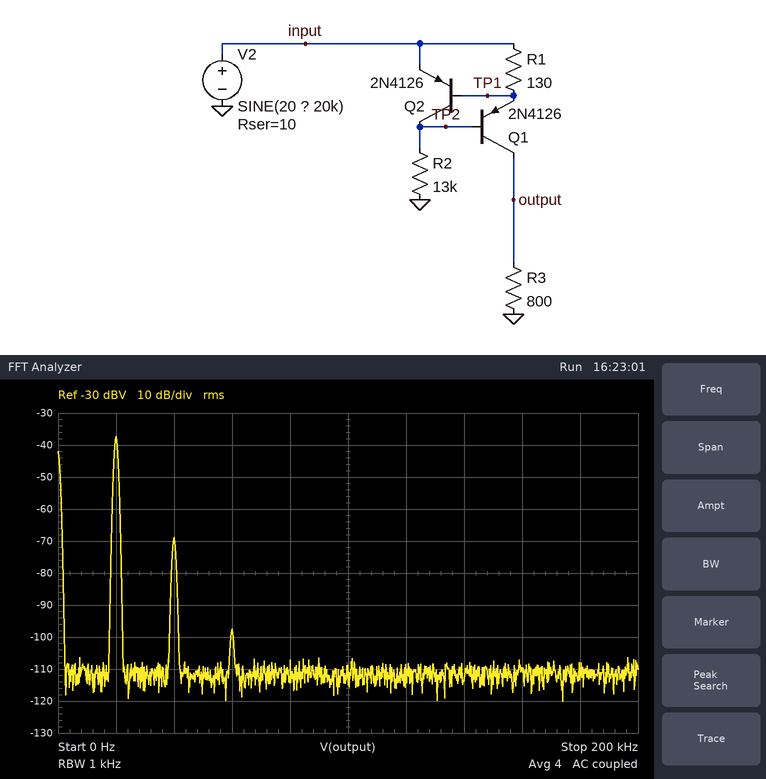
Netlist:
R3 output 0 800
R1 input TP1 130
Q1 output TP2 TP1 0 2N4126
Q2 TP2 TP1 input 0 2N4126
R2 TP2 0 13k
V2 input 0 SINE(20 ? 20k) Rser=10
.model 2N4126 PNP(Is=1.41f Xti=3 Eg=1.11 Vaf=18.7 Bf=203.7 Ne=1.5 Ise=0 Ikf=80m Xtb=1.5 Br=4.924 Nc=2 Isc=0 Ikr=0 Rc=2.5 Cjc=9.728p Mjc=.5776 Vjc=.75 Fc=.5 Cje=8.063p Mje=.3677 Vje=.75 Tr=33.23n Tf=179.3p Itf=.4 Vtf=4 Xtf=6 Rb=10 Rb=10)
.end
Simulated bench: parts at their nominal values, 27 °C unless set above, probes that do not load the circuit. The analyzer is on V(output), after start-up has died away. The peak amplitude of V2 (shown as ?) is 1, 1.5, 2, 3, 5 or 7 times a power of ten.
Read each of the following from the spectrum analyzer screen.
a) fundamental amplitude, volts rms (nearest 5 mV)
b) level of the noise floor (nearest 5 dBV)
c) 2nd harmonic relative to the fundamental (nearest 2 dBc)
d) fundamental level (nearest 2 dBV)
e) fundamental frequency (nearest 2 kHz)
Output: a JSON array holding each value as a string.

["15 mV", "-110 dBV", "-32 dBc", "-38 dBV", "20 kHz"]
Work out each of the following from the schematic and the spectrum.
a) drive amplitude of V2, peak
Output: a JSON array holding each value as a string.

["2 V"]
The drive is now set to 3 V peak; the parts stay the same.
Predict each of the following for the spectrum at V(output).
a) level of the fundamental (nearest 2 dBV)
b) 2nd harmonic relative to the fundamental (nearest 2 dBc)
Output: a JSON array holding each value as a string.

["-34 dBV", "-28 dBc"]
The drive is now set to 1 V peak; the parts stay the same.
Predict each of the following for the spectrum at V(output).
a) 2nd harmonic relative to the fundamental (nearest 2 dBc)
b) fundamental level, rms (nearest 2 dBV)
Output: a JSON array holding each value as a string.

["-38 dBc", "-44 dBV"]
